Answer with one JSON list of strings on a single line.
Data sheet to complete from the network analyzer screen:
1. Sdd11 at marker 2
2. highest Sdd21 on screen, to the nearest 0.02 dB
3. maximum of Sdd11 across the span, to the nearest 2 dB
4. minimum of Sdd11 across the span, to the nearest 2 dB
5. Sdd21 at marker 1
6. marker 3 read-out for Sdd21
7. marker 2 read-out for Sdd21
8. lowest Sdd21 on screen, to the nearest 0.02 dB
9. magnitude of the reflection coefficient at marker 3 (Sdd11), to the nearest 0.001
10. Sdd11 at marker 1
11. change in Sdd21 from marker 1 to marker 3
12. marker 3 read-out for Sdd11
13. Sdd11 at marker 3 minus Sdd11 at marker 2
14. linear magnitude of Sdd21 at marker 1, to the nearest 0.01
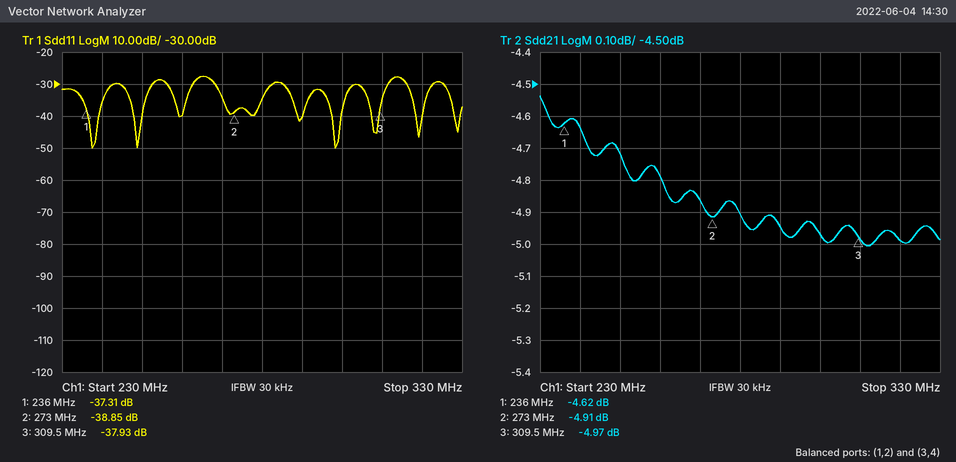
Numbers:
["-38.85 dB", "-4.54 dB", "-28 dB", "-50 dB", "-4.62 dB", "-4.97 dB", "-4.91 dB", "-5.00 dB", "0.013", "-37.31 dB", "-0.35 dB", "-37.93 dB", "0.92 dB", "0.59"]
